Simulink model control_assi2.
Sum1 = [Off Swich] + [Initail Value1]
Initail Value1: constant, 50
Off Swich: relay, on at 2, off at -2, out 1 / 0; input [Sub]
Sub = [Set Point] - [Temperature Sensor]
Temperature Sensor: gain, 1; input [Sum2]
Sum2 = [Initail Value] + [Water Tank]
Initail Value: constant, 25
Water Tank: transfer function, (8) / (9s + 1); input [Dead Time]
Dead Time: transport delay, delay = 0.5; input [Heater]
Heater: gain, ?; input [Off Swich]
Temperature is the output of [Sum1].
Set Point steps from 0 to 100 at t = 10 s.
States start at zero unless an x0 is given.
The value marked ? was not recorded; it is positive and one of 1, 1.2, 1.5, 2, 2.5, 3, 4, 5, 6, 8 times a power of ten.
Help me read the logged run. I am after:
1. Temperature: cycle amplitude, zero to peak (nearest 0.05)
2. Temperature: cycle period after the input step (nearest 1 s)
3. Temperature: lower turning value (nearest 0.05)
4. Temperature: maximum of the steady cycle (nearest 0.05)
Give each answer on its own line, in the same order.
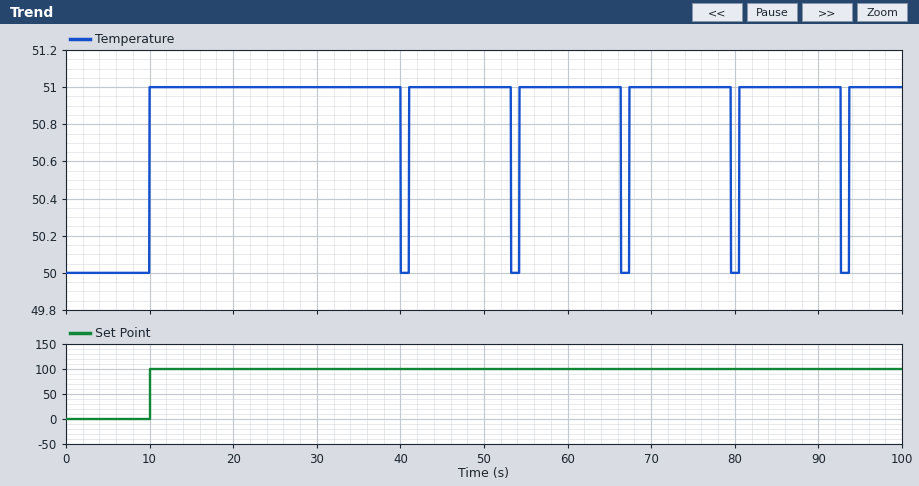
0.50
13 s
50.00
51.00
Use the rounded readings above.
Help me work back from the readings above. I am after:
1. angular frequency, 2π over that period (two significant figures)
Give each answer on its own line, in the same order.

0.48 rad/s
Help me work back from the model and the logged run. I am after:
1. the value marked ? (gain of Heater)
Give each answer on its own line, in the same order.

10
